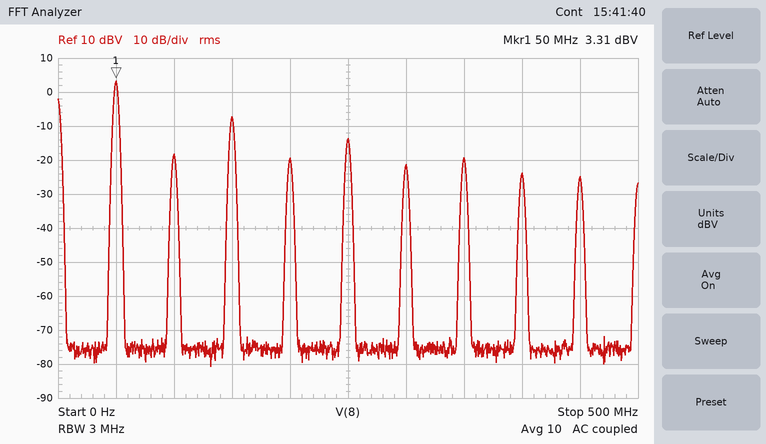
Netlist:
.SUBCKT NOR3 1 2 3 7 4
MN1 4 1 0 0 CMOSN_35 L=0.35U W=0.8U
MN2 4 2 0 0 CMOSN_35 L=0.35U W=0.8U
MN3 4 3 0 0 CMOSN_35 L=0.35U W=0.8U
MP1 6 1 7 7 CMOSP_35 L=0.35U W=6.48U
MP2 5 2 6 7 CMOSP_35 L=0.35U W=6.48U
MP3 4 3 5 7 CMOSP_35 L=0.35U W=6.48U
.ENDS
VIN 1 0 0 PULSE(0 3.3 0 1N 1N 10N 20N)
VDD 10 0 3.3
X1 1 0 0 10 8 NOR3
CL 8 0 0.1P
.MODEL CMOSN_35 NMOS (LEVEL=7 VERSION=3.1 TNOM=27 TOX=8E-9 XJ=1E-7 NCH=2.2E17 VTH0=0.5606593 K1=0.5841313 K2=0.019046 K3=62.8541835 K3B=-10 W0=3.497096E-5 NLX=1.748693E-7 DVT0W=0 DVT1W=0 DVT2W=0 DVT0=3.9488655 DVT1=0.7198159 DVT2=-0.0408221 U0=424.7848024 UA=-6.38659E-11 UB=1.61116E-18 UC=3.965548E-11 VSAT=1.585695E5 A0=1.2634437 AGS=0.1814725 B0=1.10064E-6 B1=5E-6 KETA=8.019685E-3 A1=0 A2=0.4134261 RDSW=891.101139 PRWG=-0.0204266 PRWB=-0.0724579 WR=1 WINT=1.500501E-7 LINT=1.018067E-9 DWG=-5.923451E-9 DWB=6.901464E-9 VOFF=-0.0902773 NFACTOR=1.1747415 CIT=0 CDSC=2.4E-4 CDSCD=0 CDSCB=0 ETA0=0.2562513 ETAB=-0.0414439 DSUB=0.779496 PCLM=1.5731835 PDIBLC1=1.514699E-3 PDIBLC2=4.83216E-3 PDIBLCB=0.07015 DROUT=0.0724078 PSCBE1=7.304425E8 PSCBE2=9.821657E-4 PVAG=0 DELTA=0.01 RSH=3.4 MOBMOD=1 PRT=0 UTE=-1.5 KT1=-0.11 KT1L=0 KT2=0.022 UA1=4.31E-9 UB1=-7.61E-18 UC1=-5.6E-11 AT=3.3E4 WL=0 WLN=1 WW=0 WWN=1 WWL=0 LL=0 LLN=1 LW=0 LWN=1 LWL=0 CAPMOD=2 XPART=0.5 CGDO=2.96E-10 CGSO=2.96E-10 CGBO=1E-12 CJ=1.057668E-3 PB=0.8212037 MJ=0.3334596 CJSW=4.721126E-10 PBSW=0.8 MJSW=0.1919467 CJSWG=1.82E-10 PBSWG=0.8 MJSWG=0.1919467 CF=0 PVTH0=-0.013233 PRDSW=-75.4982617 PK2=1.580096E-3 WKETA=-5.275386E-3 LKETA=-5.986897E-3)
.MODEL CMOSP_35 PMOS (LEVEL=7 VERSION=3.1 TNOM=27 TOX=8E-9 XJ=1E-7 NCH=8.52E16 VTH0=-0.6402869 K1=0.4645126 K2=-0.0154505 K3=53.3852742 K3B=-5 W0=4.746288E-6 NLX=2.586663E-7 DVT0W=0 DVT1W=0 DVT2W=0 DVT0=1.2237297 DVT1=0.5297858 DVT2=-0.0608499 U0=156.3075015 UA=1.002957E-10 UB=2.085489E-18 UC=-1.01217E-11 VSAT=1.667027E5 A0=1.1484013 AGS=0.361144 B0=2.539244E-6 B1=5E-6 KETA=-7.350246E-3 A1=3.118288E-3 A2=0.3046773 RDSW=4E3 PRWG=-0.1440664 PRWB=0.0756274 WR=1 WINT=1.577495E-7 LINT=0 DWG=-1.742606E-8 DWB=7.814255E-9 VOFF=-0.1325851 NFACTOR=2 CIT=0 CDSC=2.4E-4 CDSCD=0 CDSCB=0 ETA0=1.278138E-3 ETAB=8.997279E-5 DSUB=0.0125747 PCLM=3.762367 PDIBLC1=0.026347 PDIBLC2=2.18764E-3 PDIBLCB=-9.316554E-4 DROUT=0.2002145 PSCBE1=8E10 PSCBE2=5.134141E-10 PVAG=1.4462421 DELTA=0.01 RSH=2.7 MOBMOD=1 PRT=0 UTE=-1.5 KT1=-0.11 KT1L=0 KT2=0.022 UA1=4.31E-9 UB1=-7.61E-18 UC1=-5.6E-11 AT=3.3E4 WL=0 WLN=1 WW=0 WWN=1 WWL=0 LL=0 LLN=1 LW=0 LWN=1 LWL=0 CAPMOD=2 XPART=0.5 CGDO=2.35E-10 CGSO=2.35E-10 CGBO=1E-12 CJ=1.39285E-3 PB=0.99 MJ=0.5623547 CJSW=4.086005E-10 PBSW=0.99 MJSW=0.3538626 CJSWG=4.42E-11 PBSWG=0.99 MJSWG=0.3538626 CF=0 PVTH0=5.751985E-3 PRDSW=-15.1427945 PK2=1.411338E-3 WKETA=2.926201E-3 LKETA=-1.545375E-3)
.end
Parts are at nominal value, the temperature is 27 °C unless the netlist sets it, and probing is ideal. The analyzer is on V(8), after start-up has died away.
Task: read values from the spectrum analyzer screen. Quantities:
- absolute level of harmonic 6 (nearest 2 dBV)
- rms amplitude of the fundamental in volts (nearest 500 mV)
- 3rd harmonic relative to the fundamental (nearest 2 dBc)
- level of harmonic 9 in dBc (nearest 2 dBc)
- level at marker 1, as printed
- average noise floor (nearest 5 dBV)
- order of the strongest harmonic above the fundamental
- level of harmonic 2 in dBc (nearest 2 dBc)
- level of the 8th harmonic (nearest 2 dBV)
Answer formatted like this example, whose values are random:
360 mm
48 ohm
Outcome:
-22 dBV
1.5 V
-10 dBc
-28 dBc
3.31 dBV
-75 dBV
3
-22 dBc
-24 dBV
